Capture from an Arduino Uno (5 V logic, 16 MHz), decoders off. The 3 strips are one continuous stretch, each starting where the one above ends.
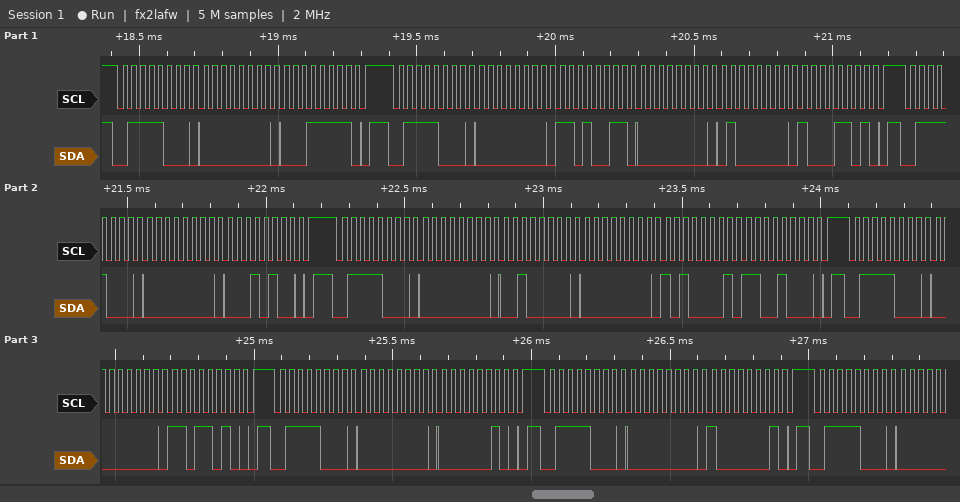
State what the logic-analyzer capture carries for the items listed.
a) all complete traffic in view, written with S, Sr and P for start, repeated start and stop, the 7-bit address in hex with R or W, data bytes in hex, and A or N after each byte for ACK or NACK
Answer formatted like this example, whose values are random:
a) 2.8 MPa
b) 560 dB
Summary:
a) S 3CW A 00 A 1F A P S 3CW A 00 A D3 A 00 A 40 A 8D A P S 3CW A 00 A 14 A P S 3CW A 00 A 20 A 00 A A1 A C8 A P S 3CW A 00 A DA A P S 3CW A 00 A 02 A P S 3CW A 00 A 81 A P S 3CW A
